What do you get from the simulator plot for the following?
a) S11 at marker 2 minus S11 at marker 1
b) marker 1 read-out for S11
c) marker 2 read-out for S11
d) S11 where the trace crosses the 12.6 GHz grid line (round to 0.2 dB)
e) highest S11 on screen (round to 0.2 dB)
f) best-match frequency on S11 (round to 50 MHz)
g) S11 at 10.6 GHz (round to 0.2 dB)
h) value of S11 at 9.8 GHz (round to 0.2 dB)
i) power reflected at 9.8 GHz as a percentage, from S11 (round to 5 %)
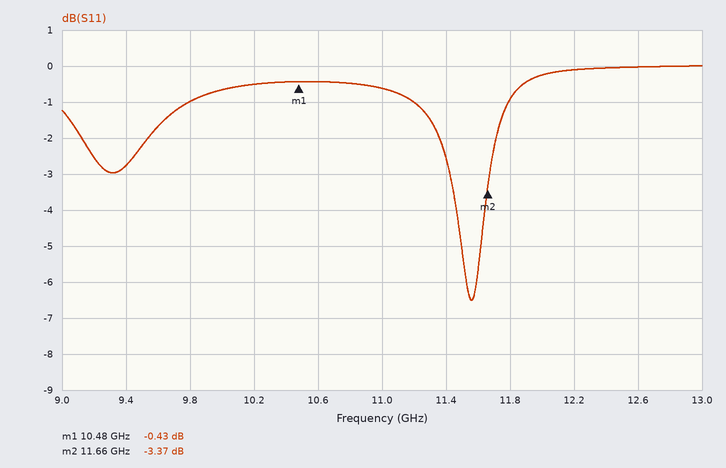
-2.94 dB
-0.43 dB
-3.37 dB
0.0 dB
0.0 dB
11.55 GHz
-0.4 dB
-1.0 dB
80 %
